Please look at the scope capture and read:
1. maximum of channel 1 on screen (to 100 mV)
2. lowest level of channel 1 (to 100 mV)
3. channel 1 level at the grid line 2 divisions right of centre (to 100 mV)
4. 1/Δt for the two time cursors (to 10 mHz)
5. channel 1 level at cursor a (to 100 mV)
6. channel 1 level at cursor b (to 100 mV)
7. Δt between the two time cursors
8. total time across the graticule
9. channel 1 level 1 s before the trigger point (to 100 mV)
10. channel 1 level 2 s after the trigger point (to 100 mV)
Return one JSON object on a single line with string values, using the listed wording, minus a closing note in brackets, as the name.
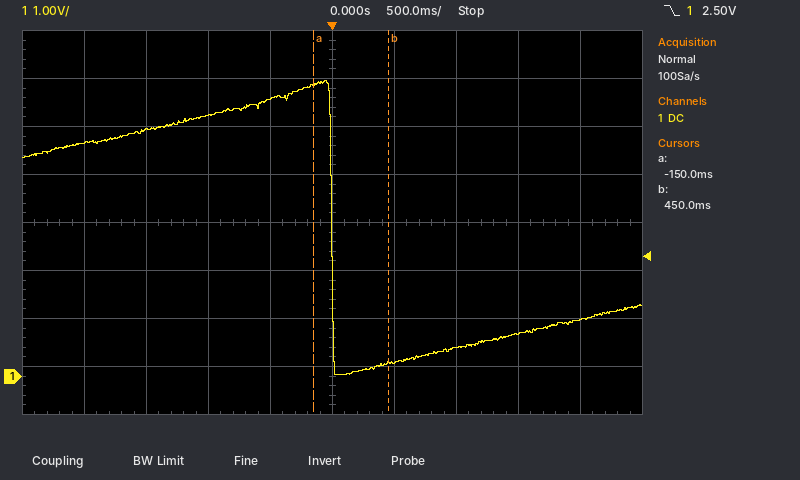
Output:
{"maximum of channel 1 on screen": "6.2 V", "lowest level of channel 1": "0.0 V", "channel 1 level at the grid line 2 divisions right of centre": "600 mV", "1/Δt for the two time cursors": "1.67 Hz", "channel 1 level at cursor a": "6.1 V", "channel 1 level at cursor b": "300 mV", "Δt between the two time cursors": "600 ms", "total time across the graticule": "5 s", "channel 1 level 1 s before the trigger point": "5.4 V", "channel 1 level 2 s after the trigger point": "1.2 V"}
